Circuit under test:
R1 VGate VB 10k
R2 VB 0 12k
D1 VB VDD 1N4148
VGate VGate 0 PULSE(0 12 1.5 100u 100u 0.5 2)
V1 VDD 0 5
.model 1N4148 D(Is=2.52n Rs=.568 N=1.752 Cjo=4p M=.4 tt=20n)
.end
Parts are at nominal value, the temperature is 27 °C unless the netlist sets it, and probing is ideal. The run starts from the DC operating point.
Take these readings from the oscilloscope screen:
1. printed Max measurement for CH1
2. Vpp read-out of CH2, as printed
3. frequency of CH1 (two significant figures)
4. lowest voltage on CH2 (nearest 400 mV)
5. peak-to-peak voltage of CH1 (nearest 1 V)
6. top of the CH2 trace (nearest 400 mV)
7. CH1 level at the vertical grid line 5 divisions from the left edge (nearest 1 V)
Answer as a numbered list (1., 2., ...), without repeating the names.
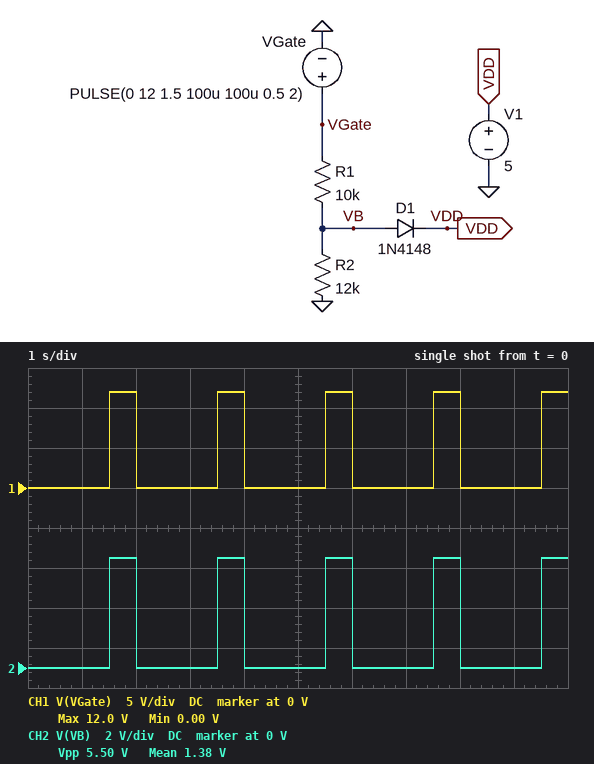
1. 12.0 V
2. 5.50 V
3. 500 mHz
4. 0 V
5. 12 V
6. 5.6 V
7. 0 V
